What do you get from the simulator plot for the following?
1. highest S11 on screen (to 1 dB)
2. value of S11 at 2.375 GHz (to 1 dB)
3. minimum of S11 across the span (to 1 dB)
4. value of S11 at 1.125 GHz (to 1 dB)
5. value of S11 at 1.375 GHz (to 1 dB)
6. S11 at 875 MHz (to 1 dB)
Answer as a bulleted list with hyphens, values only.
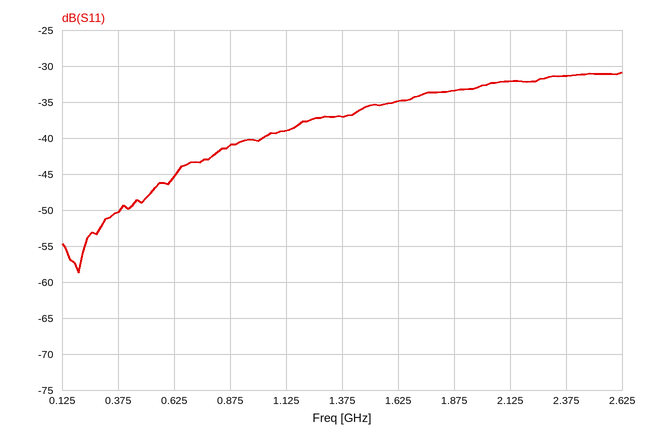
- -31 dB
- -31 dB
- -59 dB
- -39 dB
- -37 dB
- -41 dB
